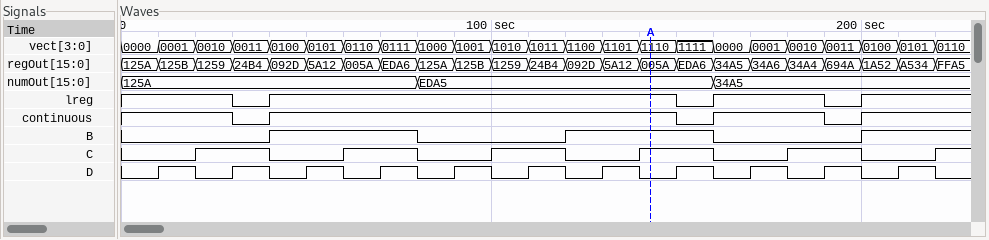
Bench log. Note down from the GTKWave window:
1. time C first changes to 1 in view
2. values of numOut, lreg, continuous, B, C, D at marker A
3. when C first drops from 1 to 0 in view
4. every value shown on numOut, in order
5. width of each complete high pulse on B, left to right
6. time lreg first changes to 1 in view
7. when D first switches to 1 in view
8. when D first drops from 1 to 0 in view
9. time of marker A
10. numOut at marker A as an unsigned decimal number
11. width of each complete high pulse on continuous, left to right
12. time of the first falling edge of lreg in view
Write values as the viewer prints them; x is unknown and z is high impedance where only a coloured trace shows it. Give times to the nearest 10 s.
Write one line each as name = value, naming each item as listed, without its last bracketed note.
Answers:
time C first changes to 1 in view = 20 s
values of numOut, lreg, continuous, B, C, D at marker A = numOut=EDA5, lreg=1, continuous=1, B=1, C=1, D=0
when C first drops from 1 to 0 in view = 40 s
every value shown on numOut, in order = 125A, EDA5, 34A5
width of each complete high pulse on B, left to right = 40 s, 40 s
time lreg first changes to 1 in view = 40 s
when D first switches to 1 in view = 10 s
when D first drops from 1 to 0 in view = 20 s
time of marker A = 140 s
numOut at marker A as an unsigned decimal number = 60837
width of each complete high pulse on continuous, left to right = 110 s, 30 s
time of the first falling edge of lreg in view = 30 s
